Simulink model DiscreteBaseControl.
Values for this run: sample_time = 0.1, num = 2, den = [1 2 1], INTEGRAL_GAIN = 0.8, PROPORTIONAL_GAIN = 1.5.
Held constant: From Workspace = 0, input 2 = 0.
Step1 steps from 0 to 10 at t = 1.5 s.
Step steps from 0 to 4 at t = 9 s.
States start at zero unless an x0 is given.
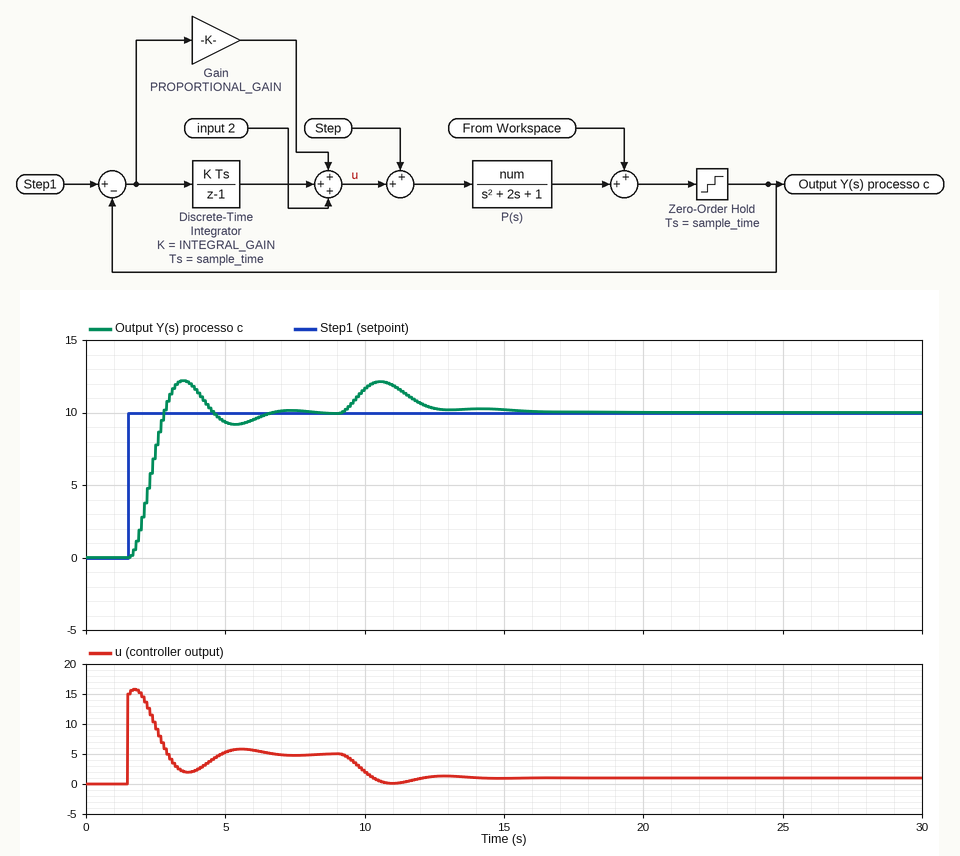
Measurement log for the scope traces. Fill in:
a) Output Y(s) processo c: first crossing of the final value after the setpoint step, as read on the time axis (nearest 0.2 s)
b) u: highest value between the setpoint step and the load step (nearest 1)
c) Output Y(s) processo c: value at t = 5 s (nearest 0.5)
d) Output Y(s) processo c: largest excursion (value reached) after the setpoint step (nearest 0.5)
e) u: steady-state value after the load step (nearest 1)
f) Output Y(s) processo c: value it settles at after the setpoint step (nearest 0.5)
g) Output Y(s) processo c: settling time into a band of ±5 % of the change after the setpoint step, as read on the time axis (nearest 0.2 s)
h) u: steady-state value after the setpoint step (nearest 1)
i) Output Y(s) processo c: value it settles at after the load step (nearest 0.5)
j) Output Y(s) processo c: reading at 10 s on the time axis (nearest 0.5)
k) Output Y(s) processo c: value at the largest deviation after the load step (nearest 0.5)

2.8 s
16
9.5
12.0
1
10.0
6.0 s
5
10.0
11.5
12.0
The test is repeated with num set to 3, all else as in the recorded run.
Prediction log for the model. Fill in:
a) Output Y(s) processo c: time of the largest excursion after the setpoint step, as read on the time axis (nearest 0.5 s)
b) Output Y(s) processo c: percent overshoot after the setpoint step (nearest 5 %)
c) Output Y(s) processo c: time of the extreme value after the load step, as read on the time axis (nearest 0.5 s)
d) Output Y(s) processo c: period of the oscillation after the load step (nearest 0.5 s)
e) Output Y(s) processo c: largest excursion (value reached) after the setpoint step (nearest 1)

3.0 s
35 %
10.5 s
3.0 s
13
